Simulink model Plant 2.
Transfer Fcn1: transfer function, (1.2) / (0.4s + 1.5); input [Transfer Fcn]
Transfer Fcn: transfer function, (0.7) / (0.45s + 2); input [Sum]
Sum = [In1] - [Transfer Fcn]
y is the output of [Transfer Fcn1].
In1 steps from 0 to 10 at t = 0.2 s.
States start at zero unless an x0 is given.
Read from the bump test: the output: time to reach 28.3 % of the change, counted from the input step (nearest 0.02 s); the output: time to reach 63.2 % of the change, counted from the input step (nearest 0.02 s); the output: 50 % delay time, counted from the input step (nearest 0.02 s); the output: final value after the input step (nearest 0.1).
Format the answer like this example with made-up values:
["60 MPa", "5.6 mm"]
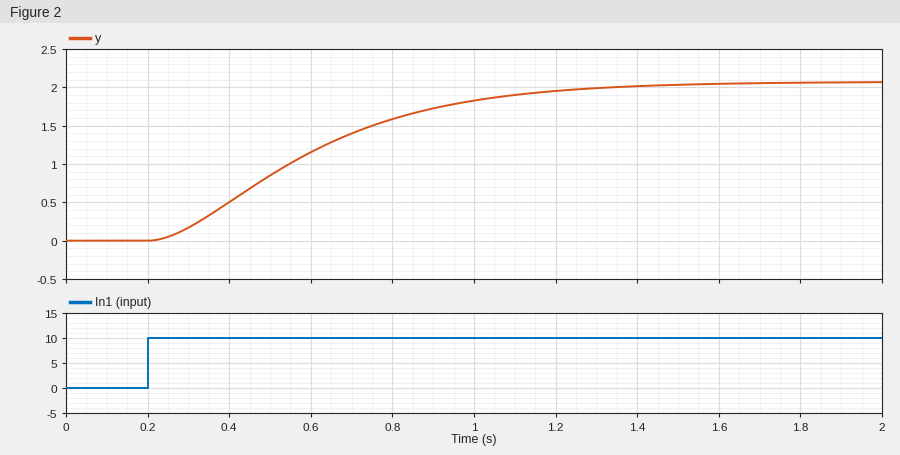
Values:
["0.22 s", "0.46 s", "0.36 s", "2.1"]
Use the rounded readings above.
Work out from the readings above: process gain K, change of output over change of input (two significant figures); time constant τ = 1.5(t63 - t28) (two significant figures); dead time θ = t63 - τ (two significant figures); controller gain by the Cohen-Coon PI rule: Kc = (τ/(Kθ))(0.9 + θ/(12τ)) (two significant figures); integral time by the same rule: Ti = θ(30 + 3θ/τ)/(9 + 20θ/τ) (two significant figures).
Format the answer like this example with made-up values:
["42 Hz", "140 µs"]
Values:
["0.21", "0.36 s", "0.10 s", "16", "0.21 s"]
